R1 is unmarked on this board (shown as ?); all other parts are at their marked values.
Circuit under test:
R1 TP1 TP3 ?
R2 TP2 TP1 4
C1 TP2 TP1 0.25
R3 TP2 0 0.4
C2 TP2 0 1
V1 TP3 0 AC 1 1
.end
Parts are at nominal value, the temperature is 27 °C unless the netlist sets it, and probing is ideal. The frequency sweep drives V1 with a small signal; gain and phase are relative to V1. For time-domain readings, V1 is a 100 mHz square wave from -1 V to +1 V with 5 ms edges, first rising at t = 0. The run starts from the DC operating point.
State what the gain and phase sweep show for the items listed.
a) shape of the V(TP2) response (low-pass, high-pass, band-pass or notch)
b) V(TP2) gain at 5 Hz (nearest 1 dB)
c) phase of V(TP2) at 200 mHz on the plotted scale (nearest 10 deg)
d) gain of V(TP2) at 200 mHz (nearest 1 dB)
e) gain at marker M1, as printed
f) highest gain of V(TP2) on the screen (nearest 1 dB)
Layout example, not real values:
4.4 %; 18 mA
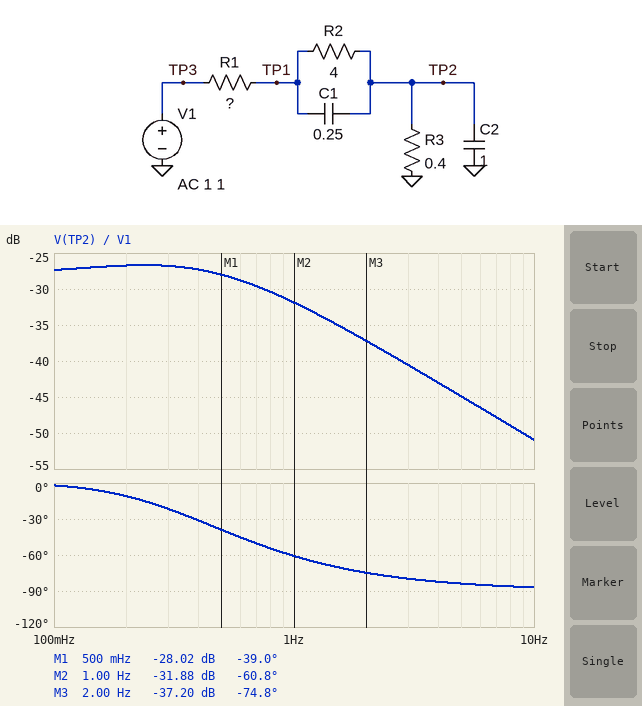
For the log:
low-pass; -45 dB; -10 deg; -27 dB; -28.02 dB; -27 dB
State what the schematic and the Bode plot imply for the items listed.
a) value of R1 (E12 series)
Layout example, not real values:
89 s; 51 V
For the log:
5.6 Ω
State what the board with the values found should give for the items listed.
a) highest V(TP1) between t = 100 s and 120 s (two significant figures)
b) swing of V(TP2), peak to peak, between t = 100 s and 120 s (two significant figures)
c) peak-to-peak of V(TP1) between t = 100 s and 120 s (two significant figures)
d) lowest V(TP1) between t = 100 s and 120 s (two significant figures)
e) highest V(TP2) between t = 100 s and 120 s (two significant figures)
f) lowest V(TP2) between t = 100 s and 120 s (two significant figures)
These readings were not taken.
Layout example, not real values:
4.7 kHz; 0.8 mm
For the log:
440 mV; 100 mV; 880 mV; -440 mV; 51 mV; -51 mV
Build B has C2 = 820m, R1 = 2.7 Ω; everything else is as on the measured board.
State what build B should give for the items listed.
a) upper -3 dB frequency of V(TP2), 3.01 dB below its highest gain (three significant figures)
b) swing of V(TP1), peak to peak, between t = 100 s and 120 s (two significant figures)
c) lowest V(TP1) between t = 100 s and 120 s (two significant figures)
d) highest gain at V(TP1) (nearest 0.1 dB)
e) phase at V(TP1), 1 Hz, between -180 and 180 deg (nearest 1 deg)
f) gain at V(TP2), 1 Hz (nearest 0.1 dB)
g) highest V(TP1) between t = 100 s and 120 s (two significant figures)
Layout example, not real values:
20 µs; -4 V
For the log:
1.04 Hz; 1.2 V; -620 mV; -4.2 dB; -62 deg; -24.6 dB; 620 mV
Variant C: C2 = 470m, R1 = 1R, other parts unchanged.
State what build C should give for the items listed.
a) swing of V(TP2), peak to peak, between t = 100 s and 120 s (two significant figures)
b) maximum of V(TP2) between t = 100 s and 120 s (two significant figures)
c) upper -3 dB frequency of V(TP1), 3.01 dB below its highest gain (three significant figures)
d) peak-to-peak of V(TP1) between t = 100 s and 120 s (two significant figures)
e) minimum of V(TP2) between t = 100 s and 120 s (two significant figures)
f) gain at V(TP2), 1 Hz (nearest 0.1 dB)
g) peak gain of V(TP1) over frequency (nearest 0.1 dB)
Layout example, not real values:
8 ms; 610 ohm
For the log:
460 mV; 230 mV; 976 mHz; 1.6 V; -230 mV; -15.3 dB; -1.8 dB
